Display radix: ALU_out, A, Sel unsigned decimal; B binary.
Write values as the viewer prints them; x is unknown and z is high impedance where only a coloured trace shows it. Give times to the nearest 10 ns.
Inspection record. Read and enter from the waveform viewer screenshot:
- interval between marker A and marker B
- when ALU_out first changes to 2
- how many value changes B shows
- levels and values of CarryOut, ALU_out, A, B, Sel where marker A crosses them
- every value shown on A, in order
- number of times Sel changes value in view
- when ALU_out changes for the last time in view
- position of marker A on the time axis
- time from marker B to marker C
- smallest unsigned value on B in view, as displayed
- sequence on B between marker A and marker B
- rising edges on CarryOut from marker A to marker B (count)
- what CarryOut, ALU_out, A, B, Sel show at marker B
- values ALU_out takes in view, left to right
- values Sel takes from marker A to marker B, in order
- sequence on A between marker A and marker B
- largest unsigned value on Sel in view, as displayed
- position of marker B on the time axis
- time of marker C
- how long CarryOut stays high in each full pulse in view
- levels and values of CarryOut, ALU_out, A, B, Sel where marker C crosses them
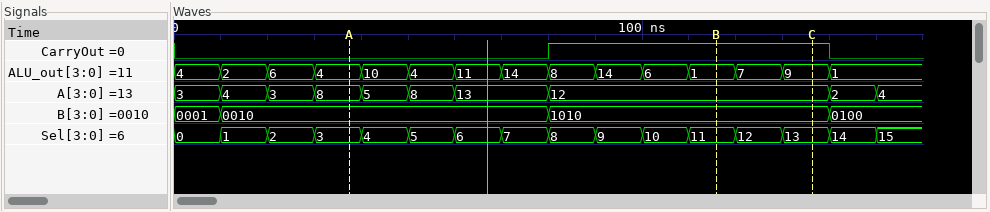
80 ns
10 ns
3
CarryOut=0, ALU_out=4, A=8, B=0010, Sel=3
3, 4, 3, 8, 5, 8, 13, 12, 2, 4
15
140 ns
40 ns
20 ns
0001
0010, 1010
1
CarryOut=1, ALU_out=1, A=12, B=1010, Sel=11
4, 2, 6, 4, 10, 4, 11, 14, 8, 14, 6, 1, 7, 9, 1
3, 4, 5, 6, 7, 8, 9, 10, 11
8, 5, 8, 13, 12
15
120 ns
140 ns
60 ns
CarryOut=1, ALU_out=9, A=12, B=1010, Sel=13
